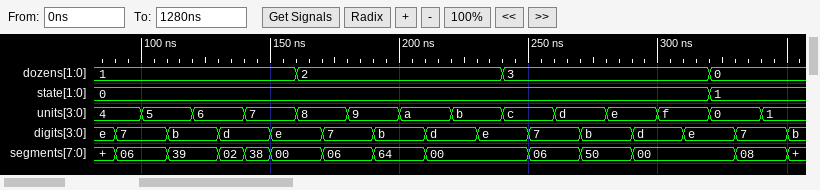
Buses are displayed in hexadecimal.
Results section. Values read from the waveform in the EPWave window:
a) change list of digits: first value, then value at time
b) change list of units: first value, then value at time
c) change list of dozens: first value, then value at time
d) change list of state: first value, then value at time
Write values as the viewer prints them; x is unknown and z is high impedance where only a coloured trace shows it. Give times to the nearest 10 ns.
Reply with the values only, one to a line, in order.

e, 7 at 90 ns, b at 110 ns, d at 130 ns, e at 150 ns, 7 at 170 ns, b at 190 ns, d at 210 ns, e at 230 ns, 7 at 250 ns, b at 270 ns, d at 290 ns, e at 310 ns, 7 at 330 ns, b at 350 ns
4, 5 at 100 ns, 6 at 120 ns, 7 at 140 ns, 8 at 160 ns, 9 at 180 ns, a at 200 ns, b at 220 ns, c at 240 ns, d at 260 ns, e at 280 ns, f at 300 ns, 0 at 320 ns, 1 at 340 ns
1, 2 at 160 ns, 3 at 240 ns, 0 at 320 ns
0, 1 at 320 ns
